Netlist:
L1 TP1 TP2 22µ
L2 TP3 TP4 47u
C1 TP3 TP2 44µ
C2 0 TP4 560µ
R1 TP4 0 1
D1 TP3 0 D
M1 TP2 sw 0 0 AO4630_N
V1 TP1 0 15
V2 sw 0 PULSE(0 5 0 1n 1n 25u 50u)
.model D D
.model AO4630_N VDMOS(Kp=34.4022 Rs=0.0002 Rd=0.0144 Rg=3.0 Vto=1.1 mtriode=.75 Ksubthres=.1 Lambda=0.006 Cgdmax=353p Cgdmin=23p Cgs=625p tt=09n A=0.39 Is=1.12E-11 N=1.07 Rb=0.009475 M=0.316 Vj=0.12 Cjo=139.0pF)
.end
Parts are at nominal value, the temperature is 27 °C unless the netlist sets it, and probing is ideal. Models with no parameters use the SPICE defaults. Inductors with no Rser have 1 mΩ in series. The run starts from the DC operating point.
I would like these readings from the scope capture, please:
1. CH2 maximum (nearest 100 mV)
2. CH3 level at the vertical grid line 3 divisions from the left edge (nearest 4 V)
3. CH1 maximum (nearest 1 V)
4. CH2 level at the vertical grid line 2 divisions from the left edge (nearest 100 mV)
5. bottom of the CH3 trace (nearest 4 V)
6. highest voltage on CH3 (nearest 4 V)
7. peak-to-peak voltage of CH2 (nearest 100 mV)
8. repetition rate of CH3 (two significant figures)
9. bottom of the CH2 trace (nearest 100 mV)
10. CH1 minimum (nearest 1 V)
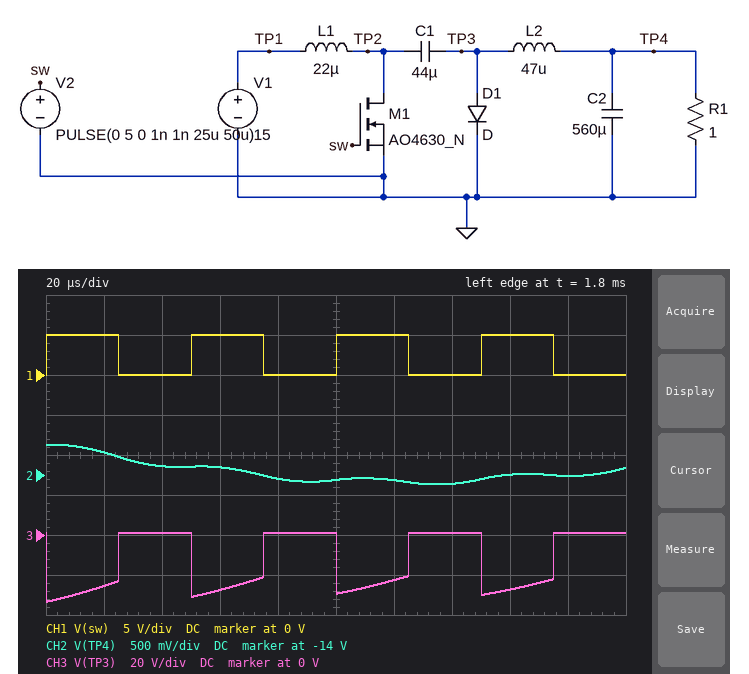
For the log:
-13.6 V
-28 V
5 V
-13.9 V
-32 V
0 V
500 mV
20 kHz
-14.1 V
0 V
